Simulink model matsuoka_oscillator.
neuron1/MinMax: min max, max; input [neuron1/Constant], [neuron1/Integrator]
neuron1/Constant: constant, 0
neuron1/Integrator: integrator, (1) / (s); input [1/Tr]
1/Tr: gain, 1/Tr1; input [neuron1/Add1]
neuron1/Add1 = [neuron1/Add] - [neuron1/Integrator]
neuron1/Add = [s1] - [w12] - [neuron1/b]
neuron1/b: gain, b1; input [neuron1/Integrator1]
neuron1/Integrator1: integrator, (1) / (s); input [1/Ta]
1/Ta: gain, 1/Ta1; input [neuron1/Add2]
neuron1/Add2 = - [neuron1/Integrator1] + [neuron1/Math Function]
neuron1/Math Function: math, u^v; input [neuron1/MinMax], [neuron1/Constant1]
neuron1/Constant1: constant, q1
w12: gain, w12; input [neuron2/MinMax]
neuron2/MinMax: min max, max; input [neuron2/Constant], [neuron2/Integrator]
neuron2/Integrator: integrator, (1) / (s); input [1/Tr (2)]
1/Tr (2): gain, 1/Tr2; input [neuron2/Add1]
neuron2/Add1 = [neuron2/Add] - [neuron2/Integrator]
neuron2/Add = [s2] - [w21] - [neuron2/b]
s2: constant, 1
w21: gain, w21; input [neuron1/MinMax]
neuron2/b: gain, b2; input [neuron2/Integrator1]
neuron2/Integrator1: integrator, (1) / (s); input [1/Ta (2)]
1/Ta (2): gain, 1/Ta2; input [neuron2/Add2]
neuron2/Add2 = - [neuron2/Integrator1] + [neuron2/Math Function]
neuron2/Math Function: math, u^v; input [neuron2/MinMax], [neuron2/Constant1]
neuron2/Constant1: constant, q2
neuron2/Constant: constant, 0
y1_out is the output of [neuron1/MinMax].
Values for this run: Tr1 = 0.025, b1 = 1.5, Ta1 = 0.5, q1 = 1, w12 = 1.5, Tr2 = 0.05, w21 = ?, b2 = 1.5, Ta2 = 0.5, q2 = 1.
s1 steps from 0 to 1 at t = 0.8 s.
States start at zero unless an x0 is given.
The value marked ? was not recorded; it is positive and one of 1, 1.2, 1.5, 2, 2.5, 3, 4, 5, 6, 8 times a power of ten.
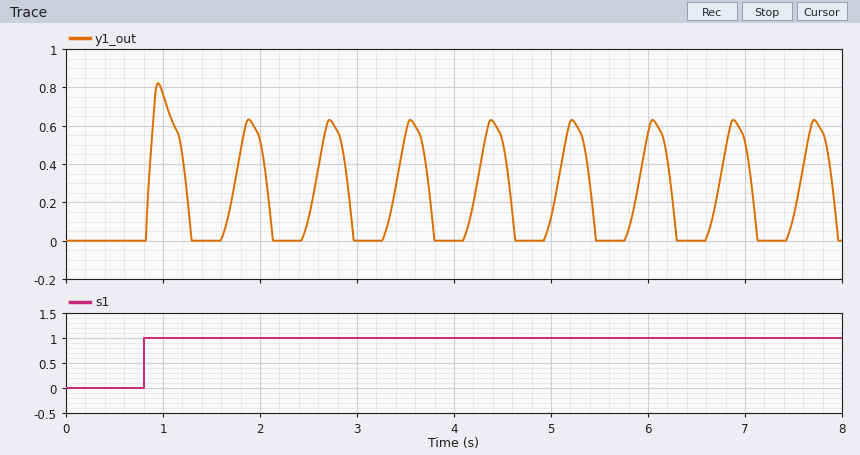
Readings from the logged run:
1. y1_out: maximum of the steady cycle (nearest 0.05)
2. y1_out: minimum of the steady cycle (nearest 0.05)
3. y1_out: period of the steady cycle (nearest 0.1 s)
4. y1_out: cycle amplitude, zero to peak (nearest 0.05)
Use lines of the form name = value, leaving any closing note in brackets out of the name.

y1_out: maximum of the steady cycle = 0.65
y1_out: minimum of the steady cycle = 0.00
y1_out: period of the steady cycle = 0.8 s
y1_out: cycle amplitude, zero to peak = 0.30
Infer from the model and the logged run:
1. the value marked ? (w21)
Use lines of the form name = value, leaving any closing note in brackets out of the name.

the value marked ? = 1
